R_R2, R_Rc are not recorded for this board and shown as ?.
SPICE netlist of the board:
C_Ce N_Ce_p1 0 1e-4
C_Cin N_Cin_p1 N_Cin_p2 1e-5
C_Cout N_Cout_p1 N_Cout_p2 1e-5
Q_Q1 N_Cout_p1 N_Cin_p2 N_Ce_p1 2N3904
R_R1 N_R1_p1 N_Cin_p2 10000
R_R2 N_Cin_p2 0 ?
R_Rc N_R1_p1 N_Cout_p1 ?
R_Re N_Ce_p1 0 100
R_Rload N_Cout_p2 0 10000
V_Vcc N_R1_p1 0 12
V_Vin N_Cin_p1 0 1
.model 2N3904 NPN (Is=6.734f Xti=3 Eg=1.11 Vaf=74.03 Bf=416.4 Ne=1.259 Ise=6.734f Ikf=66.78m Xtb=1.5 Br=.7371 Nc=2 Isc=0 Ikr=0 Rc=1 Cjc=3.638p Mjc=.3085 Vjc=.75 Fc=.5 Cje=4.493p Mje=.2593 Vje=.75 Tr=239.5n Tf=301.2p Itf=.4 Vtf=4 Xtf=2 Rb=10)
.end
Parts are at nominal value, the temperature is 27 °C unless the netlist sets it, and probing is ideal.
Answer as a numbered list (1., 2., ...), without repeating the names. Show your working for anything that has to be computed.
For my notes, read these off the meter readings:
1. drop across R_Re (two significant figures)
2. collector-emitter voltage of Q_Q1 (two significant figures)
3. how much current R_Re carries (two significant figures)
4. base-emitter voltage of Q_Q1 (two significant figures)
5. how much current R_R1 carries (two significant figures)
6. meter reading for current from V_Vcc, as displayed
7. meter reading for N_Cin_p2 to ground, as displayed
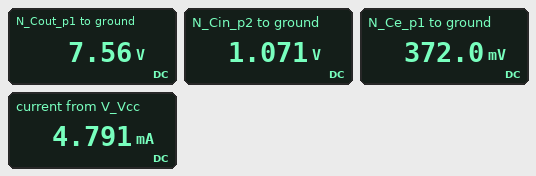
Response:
1. 372 mV = 370 mV
2. 7.56 V - 372 mV = 7.2 V
3. (372 mV) / 100 Ω = 3.7 mA
4. 1.071 V - 372 mV = 700 mV
5. (12 V - 1.071 V) / 10 kΩ = 1.1 mA
6. 4.791 mA
7. 1.071 V
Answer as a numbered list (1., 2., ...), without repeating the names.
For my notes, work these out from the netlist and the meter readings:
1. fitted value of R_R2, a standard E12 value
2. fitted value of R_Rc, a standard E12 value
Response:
1. 1 kΩ
2. 1.2 kΩ
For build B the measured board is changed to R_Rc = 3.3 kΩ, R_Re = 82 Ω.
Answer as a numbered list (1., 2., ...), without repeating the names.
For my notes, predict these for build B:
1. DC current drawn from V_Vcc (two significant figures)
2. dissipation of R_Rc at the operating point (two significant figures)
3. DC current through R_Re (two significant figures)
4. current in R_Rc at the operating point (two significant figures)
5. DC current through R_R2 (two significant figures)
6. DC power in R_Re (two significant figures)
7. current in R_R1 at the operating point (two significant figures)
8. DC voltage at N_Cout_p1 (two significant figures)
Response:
1. 4.6 mA
2. 41 mW
3. 3.6 mA
4. 3.5 mA
5. 1.0 mA
6. 1.1 mW
7. 1.1 mA
8. 410 mV
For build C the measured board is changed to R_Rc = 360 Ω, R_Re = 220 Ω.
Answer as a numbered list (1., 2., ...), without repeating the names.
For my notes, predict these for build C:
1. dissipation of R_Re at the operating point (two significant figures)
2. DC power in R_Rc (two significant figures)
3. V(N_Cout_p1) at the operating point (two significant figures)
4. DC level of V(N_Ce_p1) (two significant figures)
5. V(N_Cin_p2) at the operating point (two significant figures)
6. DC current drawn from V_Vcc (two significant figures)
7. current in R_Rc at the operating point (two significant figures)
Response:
1. 740 µW
2. 1.2 mW
3. 11 V
4. 400 mV
5. 1.1 V
6. 2.9 mA
7. 1.8 mA
